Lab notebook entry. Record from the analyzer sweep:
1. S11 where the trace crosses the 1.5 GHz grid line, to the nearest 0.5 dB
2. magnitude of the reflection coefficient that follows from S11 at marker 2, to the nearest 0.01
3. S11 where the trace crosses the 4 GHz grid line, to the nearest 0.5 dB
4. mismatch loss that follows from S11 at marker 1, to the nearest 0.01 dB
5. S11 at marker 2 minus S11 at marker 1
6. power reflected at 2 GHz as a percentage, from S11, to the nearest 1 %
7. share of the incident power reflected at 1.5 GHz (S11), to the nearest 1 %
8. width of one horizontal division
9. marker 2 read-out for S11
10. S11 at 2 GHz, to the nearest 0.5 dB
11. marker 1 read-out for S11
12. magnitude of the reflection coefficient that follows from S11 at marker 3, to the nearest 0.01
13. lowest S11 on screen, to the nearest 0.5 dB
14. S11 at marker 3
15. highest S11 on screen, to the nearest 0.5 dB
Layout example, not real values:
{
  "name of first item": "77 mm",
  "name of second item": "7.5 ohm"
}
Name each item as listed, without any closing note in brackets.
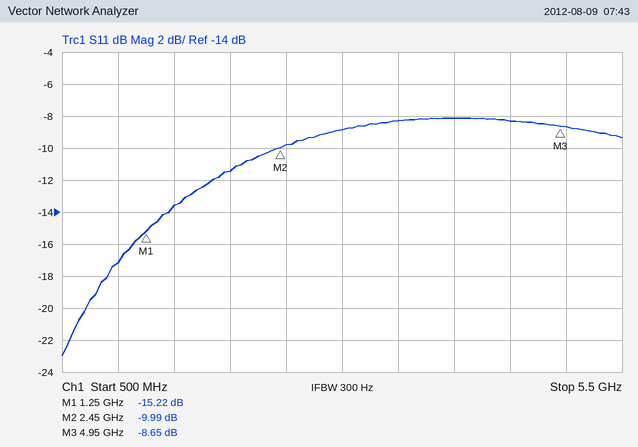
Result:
{
  "S11 where the trace crosses the 1.5 GHz grid line, to the nearest 0.5 dB": "-13.5 dB",
  "magnitude of the reflection coefficient that follows from S11 at marker 2, to the nearest 0.01": "0.32",
  "S11 where the trace crosses the 4 GHz grid line, to the nearest 0.5 dB": "-8.0 dB",
  "mismatch loss that follows from S11 at marker 1, to the nearest 0.01 dB": "0.13 dB",
  "S11 at marker 2 minus S11 at marker 1": "5.23 dB",
  "power reflected at 2 GHz as a percentage, from S11, to the nearest 1 %": "7 %",
  "share of the incident power reflected at 1.5 GHz (S11), to the nearest 1 %": "4 %",
  "width of one horizontal division": "500 MHz",
  "marker 2 read-out for S11": "-9.99 dB",
  "S11 at 2 GHz, to the nearest 0.5 dB": "-11.5 dB",
  "marker 1 read-out for S11": "-15.22 dB",
  "magnitude of the reflection coefficient that follows from S11 at marker 3, to the nearest 0.01": "0.37",
  "lowest S11 on screen, to the nearest 0.5 dB": "-23.0 dB",
  "S11 at marker 3": "-8.65 dB",
  "highest S11 on screen, to the nearest 0.5 dB": "-8.0 dB"
}
